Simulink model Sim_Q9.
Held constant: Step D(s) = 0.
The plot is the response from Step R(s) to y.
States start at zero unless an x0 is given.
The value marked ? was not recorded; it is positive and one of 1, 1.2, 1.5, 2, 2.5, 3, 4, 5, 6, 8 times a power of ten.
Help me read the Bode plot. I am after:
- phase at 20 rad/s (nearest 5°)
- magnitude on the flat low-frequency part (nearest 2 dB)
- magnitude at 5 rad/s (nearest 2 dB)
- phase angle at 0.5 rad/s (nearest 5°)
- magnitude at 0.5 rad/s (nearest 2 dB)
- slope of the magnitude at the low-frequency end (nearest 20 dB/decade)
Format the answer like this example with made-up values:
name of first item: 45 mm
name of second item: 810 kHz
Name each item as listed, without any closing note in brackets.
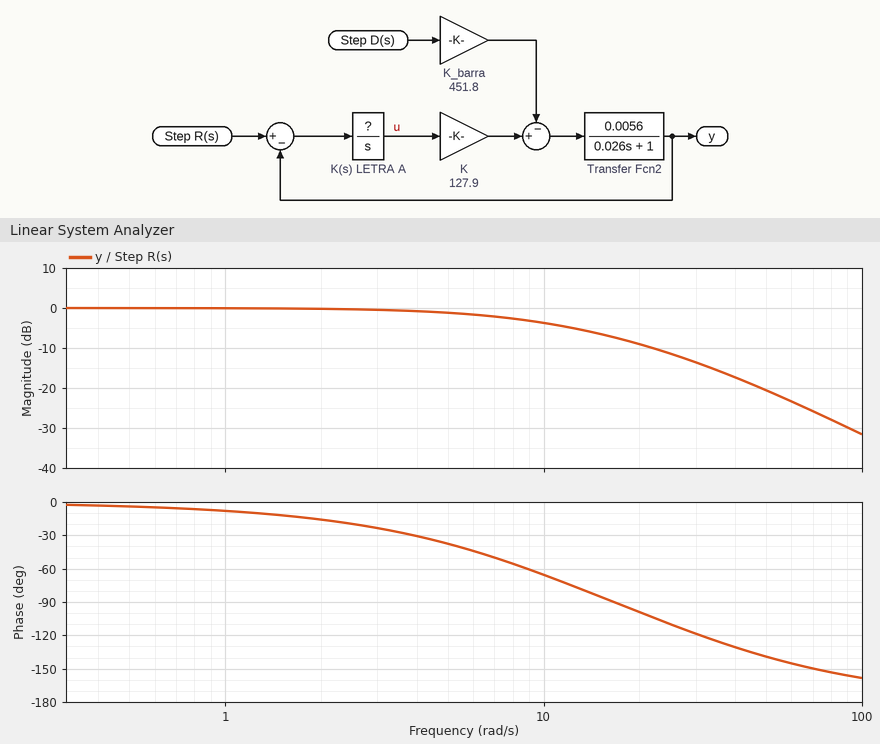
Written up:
phase at 20 rad/s: -100°
magnitude on the flat low-frequency part: 0 dB
magnitude at 5 rad/s: -2 dB
phase angle at 0.5 rad/s: -5°
magnitude at 0.5 rad/s: 0 dB
slope of the magnitude at the low-frequency end: 0 dB/decade
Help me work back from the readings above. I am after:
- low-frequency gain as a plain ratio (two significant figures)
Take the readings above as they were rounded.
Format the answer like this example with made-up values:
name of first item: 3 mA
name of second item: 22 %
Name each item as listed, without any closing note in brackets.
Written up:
low-frequency gain as a plain ratio: 1.0
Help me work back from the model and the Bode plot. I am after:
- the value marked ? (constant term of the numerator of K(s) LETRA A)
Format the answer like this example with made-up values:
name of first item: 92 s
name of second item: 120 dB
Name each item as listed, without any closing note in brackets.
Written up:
the value marked ? (constant term of the numerator of K(s) LETRA A): 10
